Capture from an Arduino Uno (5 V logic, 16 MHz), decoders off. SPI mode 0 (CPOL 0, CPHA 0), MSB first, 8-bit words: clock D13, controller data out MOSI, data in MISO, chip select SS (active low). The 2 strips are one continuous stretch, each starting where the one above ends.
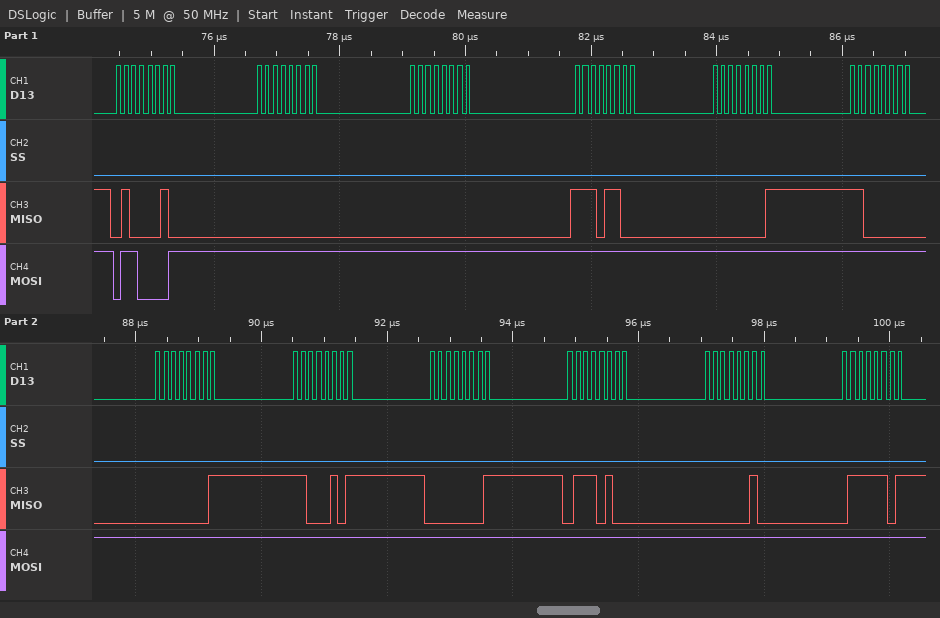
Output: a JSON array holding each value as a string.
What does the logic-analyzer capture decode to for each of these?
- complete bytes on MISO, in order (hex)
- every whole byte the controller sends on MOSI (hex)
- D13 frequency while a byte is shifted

["0x42 0x00 0x00 0xEC 0x01 0xC0 0x01 0xC5 0x01 0x74 0x02 0x7D", "0x61 0xFF 0xFF 0xFF 0xFF 0xFF 0xFF 0xFF 0xFF 0xFF 0xFF 0xFF", "8 MHz"]
